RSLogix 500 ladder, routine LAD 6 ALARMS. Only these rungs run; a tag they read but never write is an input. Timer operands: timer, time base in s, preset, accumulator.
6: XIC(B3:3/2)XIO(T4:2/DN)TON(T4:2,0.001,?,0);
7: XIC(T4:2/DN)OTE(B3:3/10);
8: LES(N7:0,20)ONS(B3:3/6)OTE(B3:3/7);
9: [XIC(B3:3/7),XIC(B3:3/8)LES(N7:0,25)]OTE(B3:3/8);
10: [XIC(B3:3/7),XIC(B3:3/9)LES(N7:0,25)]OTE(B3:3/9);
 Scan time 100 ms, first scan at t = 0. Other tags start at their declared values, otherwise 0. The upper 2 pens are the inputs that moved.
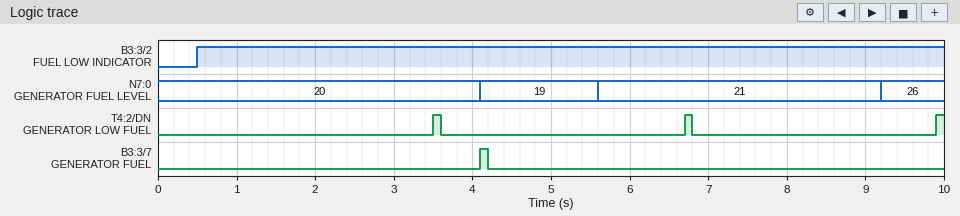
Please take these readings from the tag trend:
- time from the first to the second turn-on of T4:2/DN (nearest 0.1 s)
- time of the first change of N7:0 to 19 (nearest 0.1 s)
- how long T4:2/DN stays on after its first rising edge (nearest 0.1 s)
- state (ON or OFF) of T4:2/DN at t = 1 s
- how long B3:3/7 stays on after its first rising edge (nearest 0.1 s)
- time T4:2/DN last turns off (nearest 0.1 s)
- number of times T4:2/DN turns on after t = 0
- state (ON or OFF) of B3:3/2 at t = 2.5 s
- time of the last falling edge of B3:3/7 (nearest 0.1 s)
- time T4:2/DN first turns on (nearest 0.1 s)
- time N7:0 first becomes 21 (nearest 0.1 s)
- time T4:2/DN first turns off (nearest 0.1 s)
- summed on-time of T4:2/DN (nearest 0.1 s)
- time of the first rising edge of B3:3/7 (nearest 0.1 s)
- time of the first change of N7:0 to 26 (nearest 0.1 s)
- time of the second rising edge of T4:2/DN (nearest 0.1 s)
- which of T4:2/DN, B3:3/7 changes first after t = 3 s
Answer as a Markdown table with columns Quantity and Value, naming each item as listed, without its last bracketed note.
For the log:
| Quantity | Value |
|---|---|
| time from the first to the second turn-on of T4:2/DN | 3.2 s |
| time of the first change of N7:0 to 19 | 4.1 s |
| how long T4:2/DN stays on after its first rising edge | 0.1 s |
| state (ON or OFF) of T4:2/DN at t = 1 s | OFF |
| how long B3:3/7 stays on after its first rising edge | 0.1 s |
| time T4:2/DN last turns off | 6.8 s |
| number of times T4:2/DN turns on after t = 0 | 3 |
| state (ON or OFF) of B3:3/2 at t = 2.5 s | ON |
| time of the last falling edge of B3:3/7 | 4.2 s |
| time T4:2/DN first turns on | 3.5 s |
| time N7:0 first becomes 21 | 5.6 s |
| time T4:2/DN first turns off | 3.6 s |
| summed on-time of T4:2/DN | 0.3 s |
| time of the first rising edge of B3:3/7 | 4.1 s |
| time of the first change of N7:0 to 26 | 9.2 s |
| time of the second rising edge of T4:2/DN | 6.7 s |
| which of T4:2/DN, B3:3/7 changes first after t = 3 s | T4:2/DN |
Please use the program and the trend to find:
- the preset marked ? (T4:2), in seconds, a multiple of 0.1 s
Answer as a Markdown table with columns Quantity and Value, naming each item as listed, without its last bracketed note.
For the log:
| Quantity | Value |
|---|---|
| the preset marked ? (T4:2), in seconds, a multiple of 0.1 s | 3.0 s |
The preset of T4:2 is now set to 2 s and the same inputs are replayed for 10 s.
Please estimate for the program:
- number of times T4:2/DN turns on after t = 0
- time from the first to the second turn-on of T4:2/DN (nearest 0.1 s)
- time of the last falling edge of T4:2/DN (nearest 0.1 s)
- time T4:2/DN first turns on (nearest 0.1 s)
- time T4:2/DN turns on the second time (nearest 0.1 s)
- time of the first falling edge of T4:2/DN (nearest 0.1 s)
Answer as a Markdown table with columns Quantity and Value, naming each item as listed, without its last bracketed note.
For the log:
| Quantity | Value |
|---|---|
| number of times T4:2/DN turns on after t = 0 | 4 |
| time from the first to the second turn-on of T4:2/DN | 2.2 s |
| time of the last falling edge of T4:2/DN | 9.2 s |
| time T4:2/DN first turns on | 2.5 s |
| time T4:2/DN turns on the second time | 4.7 s |
| time of the first falling edge of T4:2/DN | 2.6 s |
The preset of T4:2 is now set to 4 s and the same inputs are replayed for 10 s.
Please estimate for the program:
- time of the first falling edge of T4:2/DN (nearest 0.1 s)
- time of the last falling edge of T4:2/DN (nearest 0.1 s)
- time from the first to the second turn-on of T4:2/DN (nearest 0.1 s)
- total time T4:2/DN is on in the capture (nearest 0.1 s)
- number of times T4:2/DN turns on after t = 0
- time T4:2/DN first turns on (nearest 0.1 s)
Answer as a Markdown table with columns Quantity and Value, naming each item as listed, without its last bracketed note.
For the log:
| Quantity | Value |
|---|---|
| time of the first falling edge of T4:2/DN | 4.6 s |
| time of the last falling edge of T4:2/DN | 8.8 s |
| time from the first to the second turn-on of T4:2/DN | 4.2 s |
| total time T4:2/DN is on in the capture | 0.2 s |
| number of times T4:2/DN turns on after t = 0 | 2 |
| time T4:2/DN first turns on | 4.5 s |
